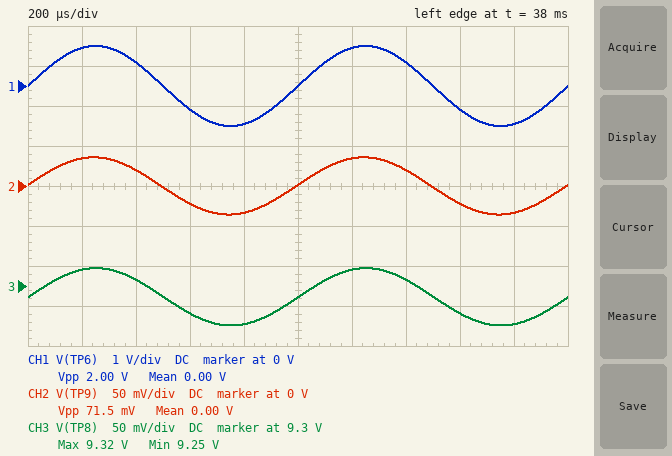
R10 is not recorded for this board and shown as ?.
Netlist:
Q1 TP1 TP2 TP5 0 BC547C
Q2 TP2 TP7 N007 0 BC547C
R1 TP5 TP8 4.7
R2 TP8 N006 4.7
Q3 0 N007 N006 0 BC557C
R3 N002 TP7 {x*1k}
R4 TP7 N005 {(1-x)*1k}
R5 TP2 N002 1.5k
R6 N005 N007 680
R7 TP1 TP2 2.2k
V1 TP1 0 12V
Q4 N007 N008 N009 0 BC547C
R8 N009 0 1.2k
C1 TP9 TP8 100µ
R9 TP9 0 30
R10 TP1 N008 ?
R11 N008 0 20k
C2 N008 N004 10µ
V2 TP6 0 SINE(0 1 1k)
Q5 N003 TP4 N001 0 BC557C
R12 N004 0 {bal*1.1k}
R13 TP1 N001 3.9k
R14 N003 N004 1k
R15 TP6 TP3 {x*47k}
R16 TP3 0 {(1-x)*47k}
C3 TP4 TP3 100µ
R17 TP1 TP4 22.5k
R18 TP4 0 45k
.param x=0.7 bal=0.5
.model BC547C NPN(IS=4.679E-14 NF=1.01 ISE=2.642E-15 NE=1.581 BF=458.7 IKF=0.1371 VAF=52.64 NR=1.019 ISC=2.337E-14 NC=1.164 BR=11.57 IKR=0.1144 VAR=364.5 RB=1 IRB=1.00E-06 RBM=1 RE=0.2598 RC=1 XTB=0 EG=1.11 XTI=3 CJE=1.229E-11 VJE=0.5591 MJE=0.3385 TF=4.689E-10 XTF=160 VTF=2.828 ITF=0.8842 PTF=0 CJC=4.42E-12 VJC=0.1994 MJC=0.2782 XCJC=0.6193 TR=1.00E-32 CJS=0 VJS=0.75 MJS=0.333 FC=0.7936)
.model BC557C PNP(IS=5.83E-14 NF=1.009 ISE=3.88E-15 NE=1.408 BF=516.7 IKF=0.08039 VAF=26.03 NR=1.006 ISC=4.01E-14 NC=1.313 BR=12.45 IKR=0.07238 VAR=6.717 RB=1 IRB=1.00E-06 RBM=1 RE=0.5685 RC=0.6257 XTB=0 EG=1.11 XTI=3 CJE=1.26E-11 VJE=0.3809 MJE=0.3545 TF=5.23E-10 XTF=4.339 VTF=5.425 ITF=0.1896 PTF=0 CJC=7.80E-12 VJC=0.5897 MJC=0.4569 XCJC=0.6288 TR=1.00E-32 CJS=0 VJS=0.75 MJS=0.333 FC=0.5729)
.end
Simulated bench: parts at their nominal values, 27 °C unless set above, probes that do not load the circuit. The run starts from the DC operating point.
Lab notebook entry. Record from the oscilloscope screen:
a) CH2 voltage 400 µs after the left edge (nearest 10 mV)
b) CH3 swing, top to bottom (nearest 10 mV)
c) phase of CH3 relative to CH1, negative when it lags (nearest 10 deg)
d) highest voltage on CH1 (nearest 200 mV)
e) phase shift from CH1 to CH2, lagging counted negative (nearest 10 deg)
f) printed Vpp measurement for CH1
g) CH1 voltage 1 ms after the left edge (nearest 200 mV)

20 mV
70 mV
0 deg
1.0 V
0 deg
2.00 V
0 V
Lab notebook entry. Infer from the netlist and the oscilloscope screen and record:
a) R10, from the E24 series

130 kΩ
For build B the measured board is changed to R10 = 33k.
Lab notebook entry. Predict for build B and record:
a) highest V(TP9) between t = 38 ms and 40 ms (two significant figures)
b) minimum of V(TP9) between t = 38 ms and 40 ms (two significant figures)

2.1 mV
-1.5 mV
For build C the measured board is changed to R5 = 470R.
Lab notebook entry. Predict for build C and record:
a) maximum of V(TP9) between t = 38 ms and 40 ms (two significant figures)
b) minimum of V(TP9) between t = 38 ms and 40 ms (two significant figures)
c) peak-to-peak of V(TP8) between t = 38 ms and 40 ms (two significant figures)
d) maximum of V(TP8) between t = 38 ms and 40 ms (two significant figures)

30 mV
-31 mV
61 mV
9.6 V
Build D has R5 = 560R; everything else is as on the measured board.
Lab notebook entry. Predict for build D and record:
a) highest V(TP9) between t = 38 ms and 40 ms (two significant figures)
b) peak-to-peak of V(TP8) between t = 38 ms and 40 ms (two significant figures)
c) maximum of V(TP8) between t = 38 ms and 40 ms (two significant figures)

33 mV
67 mV
9.6 V
